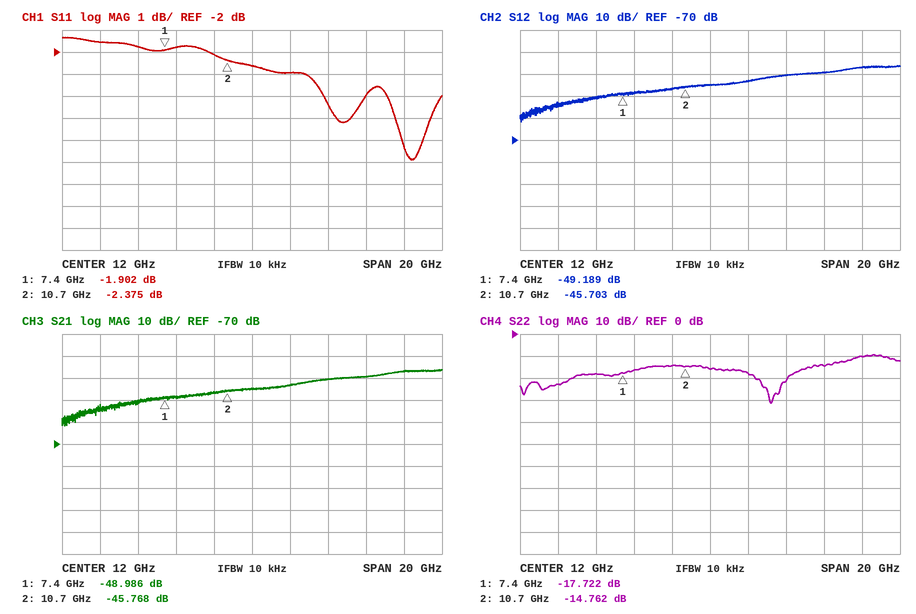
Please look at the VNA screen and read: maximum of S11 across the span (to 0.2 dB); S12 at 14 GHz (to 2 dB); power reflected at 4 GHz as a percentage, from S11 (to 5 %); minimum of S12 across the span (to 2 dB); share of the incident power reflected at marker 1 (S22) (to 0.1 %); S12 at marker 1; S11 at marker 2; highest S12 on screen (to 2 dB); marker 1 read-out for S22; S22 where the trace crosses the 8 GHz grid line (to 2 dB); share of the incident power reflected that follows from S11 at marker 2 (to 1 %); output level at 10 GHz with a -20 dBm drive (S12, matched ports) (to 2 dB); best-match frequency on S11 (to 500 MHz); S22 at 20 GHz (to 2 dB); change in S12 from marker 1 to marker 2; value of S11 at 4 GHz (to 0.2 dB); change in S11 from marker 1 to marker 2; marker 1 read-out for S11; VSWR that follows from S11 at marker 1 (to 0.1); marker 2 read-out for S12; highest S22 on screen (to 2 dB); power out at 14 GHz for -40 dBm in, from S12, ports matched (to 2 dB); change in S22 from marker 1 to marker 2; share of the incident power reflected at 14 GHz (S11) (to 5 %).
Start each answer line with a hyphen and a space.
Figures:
- -1.4 dB
- -44 dB
- 70 %
- -62 dB
- 1.7 %
- -49.189 dB
- -2.375 dB
- -36 dB
- -17.722 dB
- -16 dB
- 58 %
- -66 dBm
- 20.5 GHz
- -10 dB
- 3.486 dB
- -1.6 dB
- -0.473 dB
- -1.902 dB
- 9.2
- -45.703 dB
- -10 dB
- -84 dBm
- 2.960 dB
- 50 %
